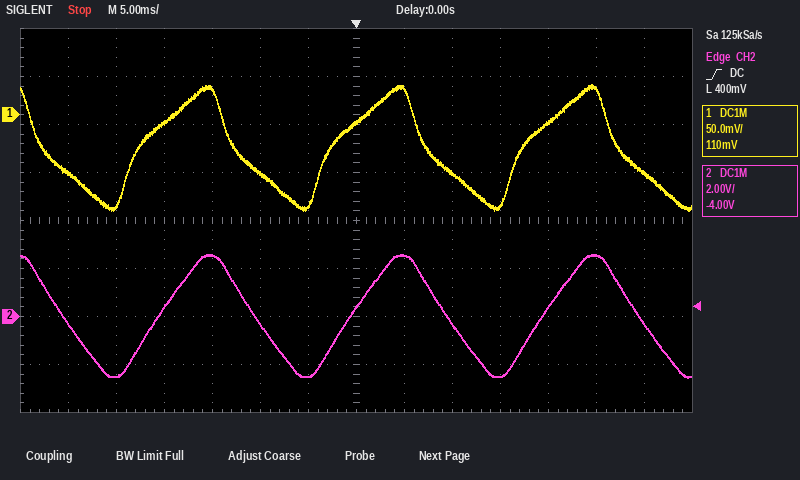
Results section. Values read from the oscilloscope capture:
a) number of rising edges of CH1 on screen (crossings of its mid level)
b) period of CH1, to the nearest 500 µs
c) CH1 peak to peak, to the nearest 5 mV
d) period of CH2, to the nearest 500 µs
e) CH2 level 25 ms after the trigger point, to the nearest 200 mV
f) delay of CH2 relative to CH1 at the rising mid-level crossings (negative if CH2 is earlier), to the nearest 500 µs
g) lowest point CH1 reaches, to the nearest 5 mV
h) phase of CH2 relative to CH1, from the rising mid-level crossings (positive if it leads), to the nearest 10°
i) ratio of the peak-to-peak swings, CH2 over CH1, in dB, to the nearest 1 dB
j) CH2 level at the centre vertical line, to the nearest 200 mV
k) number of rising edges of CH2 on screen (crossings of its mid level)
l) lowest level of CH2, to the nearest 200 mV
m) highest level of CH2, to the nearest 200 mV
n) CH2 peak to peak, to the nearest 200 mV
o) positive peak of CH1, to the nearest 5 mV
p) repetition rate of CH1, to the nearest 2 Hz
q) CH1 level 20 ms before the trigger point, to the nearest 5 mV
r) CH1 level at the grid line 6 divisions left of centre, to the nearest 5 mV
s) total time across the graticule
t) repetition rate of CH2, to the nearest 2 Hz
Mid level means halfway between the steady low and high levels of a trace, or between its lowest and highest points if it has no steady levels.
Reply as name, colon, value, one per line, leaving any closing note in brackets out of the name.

number of rising edges of CH1 on screen: 3
period of CH1, to the nearest 500 µs: 20.0 ms
CH1 peak to peak, to the nearest 5 mV: 130 mV
period of CH2, to the nearest 500 µs: 20.0 ms
CH2 level 25 ms after the trigger point, to the nearest 200 mV: 2.6 V
delay of CH2 relative to CH1 at the rising mid-level crossings (negative if CH2 is earlier), to the nearest 500 µs: +2.0 ms
lowest point CH1 reaches, to the nearest 5 mV: -100 mV
phase of CH2 relative to CH1, from the rising mid-level crossings (positive if it leads), to the nearest 10°: -40°
ratio of the peak-to-peak swings, CH2 over CH1, in dB, to the nearest 1 dB: 32 dB
CH2 level at the centre vertical line, to the nearest 200 mV: 400 mV
number of rising edges of CH2 on screen: 3
lowest level of CH2, to the nearest 200 mV: -2.6 V
highest level of CH2, to the nearest 200 mV: 2.6 V
CH2 peak to peak, to the nearest 200 mV: 5.2 V
positive peak of CH1, to the nearest 5 mV: 30 mV
repetition rate of CH1, to the nearest 2 Hz: 50 Hz
CH1 level 20 ms before the trigger point, to the nearest 5 mV: -10 mV
CH1 level at the grid line 6 divisions left of centre, to the nearest 5 mV: -60 mV
total time across the graticule: 70 ms
repetition rate of CH2, to the nearest 2 Hz: 50 Hz
